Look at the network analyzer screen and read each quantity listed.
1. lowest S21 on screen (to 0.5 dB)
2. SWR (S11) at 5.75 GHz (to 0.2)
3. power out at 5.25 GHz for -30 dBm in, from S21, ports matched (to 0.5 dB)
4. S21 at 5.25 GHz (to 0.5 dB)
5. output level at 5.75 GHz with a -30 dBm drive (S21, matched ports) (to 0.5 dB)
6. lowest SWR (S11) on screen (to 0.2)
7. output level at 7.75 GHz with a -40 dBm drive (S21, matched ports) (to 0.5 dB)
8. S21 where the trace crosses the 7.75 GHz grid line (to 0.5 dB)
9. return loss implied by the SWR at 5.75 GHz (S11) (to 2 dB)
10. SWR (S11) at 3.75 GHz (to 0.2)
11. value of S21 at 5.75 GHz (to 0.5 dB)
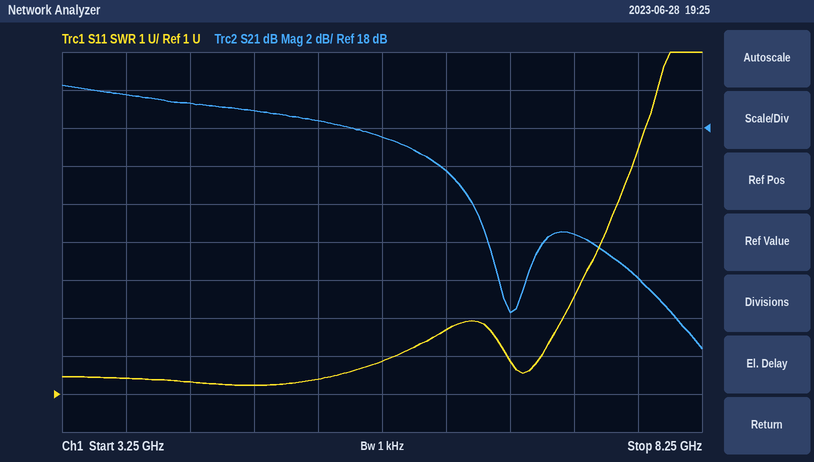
6.5 dB
1.8
-11.5 dBm
18.5 dB
-12.5 dBm
1.2
-30.0 dBm
10.0 dB
10 dB
1.4
17.5 dB
